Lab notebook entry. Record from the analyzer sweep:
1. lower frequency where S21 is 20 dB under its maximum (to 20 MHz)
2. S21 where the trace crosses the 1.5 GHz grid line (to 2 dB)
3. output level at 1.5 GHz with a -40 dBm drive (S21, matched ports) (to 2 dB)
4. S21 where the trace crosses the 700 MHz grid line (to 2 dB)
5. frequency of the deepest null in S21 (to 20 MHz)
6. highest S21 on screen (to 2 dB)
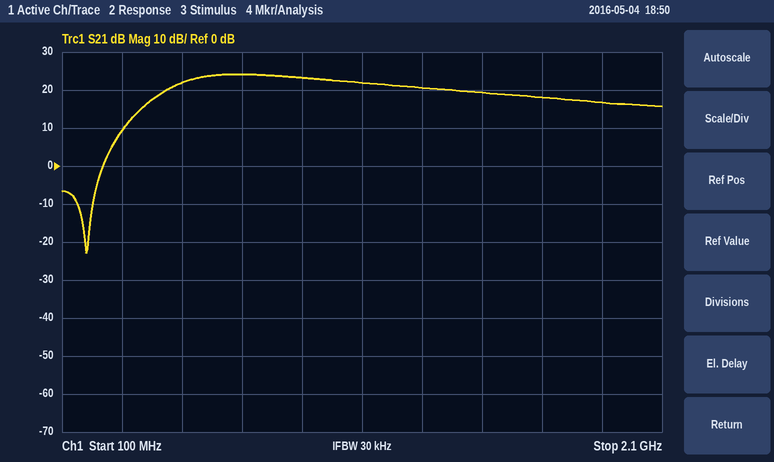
260 MHz
20 dB
-20 dBm
24 dB
180 MHz
24 dB
